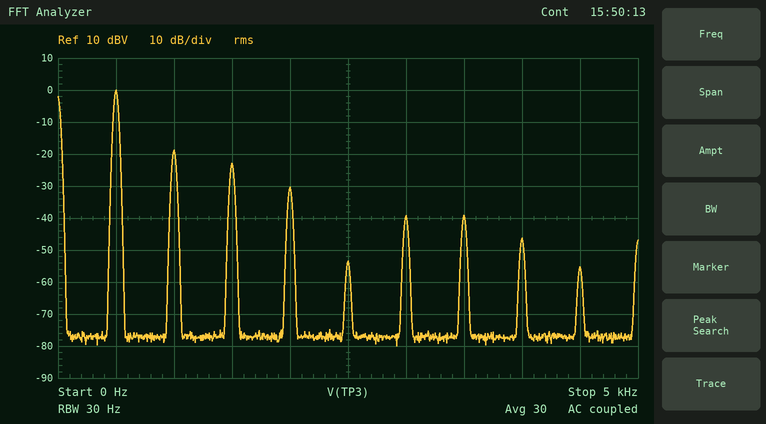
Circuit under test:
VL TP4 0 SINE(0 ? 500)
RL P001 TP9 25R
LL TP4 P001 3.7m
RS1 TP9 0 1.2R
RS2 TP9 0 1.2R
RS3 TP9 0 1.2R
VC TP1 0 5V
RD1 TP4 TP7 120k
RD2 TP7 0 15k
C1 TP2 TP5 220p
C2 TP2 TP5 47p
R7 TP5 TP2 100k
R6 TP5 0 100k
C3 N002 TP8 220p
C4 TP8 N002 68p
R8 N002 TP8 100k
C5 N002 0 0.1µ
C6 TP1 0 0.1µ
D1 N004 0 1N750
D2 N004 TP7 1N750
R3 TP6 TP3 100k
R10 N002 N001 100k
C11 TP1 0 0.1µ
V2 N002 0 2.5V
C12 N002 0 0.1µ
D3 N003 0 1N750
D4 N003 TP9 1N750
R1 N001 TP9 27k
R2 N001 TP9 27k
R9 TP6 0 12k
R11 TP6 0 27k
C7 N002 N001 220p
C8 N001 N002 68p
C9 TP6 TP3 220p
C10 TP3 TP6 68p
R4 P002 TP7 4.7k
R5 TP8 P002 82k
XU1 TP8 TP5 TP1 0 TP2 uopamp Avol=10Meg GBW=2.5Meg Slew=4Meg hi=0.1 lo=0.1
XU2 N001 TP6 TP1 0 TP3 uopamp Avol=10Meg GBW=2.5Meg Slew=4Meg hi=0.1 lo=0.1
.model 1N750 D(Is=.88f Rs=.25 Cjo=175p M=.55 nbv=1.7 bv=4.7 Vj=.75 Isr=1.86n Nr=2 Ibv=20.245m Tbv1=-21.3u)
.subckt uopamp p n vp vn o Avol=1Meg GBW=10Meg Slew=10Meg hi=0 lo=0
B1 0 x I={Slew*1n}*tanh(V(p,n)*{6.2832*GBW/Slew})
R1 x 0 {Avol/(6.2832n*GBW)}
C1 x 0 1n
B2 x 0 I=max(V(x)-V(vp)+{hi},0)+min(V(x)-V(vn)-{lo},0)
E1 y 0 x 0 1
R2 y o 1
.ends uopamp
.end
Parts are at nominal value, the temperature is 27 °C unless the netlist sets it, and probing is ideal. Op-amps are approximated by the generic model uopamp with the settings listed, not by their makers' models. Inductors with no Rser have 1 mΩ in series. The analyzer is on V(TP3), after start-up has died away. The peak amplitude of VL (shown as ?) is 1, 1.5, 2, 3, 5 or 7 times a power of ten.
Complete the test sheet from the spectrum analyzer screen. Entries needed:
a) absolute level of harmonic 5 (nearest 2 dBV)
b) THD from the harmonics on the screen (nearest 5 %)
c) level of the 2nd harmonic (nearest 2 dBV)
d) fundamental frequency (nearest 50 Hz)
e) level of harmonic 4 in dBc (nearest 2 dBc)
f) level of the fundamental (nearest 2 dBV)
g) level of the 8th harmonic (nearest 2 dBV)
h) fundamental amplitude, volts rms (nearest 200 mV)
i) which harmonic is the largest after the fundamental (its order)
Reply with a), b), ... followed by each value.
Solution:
a) -54 dBV
b) 15 %
c) -18 dBV
d) 500 Hz
e) -30 dBc
f) 0 dBV
g) -46 dBV
h) 1.0 V
i) 2
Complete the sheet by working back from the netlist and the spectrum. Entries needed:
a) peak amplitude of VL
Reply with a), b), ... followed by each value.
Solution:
a) 10 V
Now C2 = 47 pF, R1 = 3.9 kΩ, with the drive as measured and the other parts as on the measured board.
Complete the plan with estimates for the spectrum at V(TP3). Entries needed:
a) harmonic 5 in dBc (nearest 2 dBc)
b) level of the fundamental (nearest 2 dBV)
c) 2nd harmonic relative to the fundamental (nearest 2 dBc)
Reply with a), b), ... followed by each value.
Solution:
a) -40 dBc
b) 0 dBV
c) -16 dBc
